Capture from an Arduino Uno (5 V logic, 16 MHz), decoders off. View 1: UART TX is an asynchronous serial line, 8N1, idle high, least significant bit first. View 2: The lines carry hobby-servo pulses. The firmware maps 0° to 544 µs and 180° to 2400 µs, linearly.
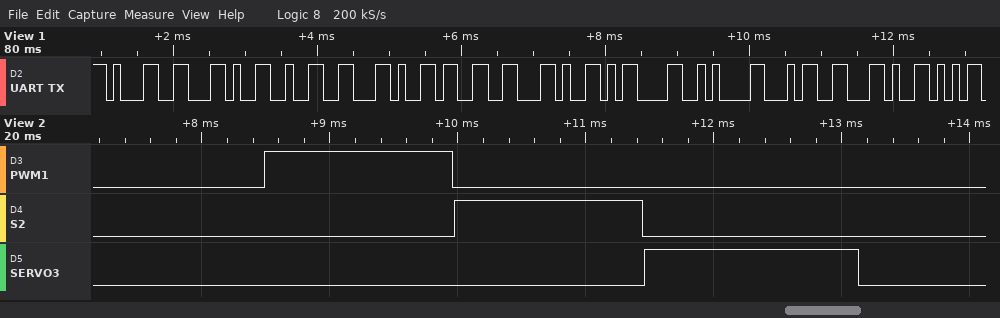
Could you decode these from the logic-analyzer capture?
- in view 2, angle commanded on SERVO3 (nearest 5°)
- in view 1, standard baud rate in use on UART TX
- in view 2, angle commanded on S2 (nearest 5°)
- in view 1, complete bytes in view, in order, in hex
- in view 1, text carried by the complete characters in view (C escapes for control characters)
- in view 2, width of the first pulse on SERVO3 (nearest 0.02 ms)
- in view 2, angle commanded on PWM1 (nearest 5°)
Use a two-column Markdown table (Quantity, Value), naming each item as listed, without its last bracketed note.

| Quantity | Value |
|---|---|
| in view 2, angle commanded on SERVO3 | 110° |
| in view 1, standard baud rate in use on UART TX | 9600 baud |
| in view 2, angle commanded on S2 | 90° |
| in view 1, complete bytes in view, in order, in hex | 31 2C 32 2C 33 2C 0D 0A 34 2C |
| in view 1, text carried by the complete characters in view | "1,2,3,\r\n4," |
| in view 2, width of the first pulse on SERVO3 | 1.68 ms |
| in view 2, angle commanded on PWM1 | 90° |
